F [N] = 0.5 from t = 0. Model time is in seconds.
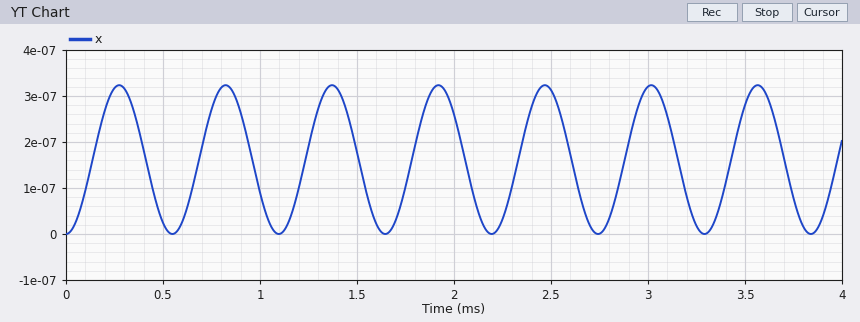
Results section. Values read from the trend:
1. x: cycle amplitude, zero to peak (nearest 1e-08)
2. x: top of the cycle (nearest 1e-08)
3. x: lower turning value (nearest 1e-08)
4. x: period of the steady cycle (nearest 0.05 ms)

0.00000016
0.00000032
0.00000000
0.55 ms
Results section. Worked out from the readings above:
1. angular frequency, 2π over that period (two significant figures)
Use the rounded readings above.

11 rad/ms
